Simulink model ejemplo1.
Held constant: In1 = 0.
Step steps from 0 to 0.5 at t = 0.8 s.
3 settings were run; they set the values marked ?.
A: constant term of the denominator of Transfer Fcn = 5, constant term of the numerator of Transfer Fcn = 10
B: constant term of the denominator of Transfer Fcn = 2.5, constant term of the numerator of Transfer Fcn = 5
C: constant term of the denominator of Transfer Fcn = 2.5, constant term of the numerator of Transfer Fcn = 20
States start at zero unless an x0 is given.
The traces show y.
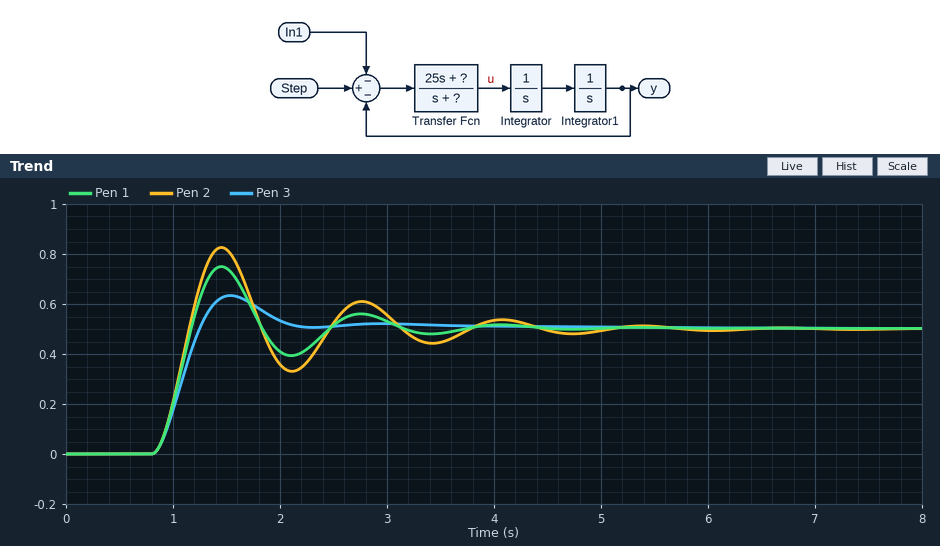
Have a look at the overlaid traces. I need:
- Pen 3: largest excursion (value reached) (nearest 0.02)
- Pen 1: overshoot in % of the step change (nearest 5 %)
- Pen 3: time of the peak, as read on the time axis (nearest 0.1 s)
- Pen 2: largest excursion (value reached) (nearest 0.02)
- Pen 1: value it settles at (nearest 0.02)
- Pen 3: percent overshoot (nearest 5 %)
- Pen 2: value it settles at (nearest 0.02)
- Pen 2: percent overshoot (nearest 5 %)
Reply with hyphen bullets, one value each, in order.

- 0.64
- 50 %
- 1.5 s
- 0.82
- 0.50
- 25 %
- 0.50
- 65 %
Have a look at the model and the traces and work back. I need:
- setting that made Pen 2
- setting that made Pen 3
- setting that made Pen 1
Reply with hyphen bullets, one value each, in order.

- C
- A
- B
